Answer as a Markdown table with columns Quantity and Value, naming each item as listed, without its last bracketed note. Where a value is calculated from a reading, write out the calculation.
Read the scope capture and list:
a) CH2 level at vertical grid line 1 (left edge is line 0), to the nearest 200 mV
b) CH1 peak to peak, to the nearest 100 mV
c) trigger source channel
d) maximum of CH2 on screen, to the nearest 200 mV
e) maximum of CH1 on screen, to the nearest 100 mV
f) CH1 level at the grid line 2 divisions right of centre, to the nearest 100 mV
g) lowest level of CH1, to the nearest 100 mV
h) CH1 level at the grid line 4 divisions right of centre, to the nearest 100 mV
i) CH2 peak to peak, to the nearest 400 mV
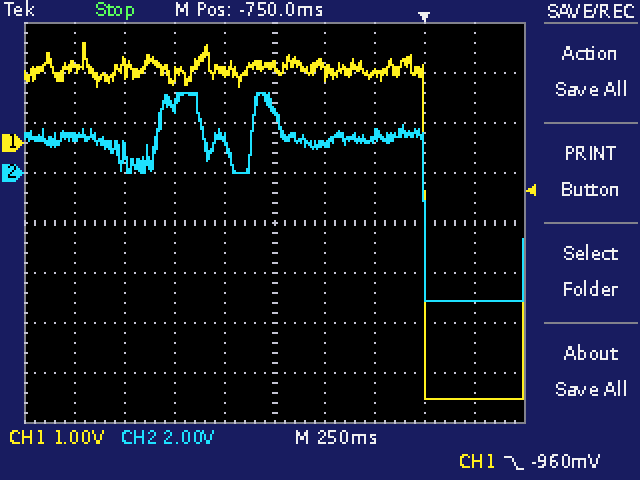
| Quantity | Value |
|---|---|
| CH2 level at vertical grid line 1 (left edge is line 0), to the nearest 200 mV | 1.4 V |
| CH1 peak to peak, to the nearest 100 mV | 2.0 V − (-5.1 V) = 7.1 V |
| trigger source channel | CH1 |
| maximum of CH2 on screen, to the nearest 200 mV | 3.2 V |
| maximum of CH1 on screen, to the nearest 100 mV | 2.0 V |
| CH1 level at the grid line 2 divisions right of centre, to the nearest 100 mV | 1.4 V |
| lowest level of CH1, to the nearest 100 mV | -5.1 V |
| CH1 level at the grid line 4 divisions right of centre, to the nearest 100 mV | -5.1 V |
| CH2 peak to peak, to the nearest 400 mV | 8.4 V |
